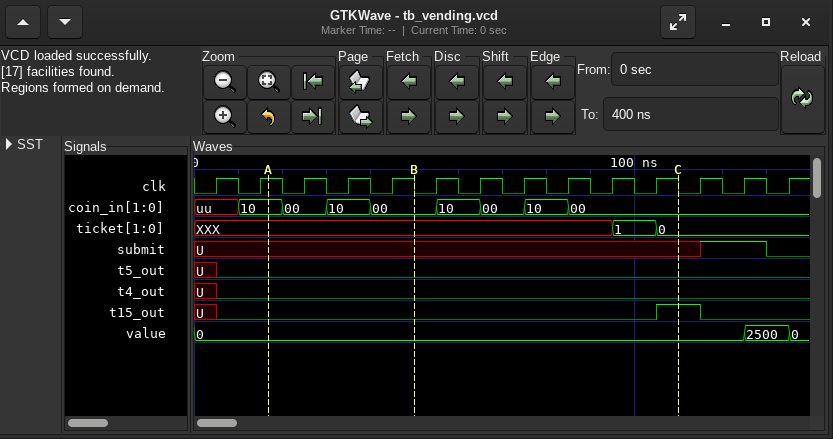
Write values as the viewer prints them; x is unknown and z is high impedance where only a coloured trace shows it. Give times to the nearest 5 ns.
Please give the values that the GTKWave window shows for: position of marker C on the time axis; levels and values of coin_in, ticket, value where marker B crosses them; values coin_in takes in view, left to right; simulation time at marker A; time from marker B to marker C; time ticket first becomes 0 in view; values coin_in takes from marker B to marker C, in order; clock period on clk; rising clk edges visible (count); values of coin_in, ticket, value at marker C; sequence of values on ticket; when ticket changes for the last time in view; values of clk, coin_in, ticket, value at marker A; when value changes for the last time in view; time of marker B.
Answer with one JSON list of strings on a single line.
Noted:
["110 ns", "coin_in=00, ticket=XXX, value=0", "uu, 10, 00, 10, 00, 10, 00, 10, 00", "15 ns", "60 ns", "105 ns", "00, 10, 00, 10, 00", "10 ns", "14", "coin_in=00, ticket=0, value=0", "XXX, 1, 0", "105 ns", "clk=1, coin_in=10, ticket=XXX, value=0", "135 ns", "50 ns"]
